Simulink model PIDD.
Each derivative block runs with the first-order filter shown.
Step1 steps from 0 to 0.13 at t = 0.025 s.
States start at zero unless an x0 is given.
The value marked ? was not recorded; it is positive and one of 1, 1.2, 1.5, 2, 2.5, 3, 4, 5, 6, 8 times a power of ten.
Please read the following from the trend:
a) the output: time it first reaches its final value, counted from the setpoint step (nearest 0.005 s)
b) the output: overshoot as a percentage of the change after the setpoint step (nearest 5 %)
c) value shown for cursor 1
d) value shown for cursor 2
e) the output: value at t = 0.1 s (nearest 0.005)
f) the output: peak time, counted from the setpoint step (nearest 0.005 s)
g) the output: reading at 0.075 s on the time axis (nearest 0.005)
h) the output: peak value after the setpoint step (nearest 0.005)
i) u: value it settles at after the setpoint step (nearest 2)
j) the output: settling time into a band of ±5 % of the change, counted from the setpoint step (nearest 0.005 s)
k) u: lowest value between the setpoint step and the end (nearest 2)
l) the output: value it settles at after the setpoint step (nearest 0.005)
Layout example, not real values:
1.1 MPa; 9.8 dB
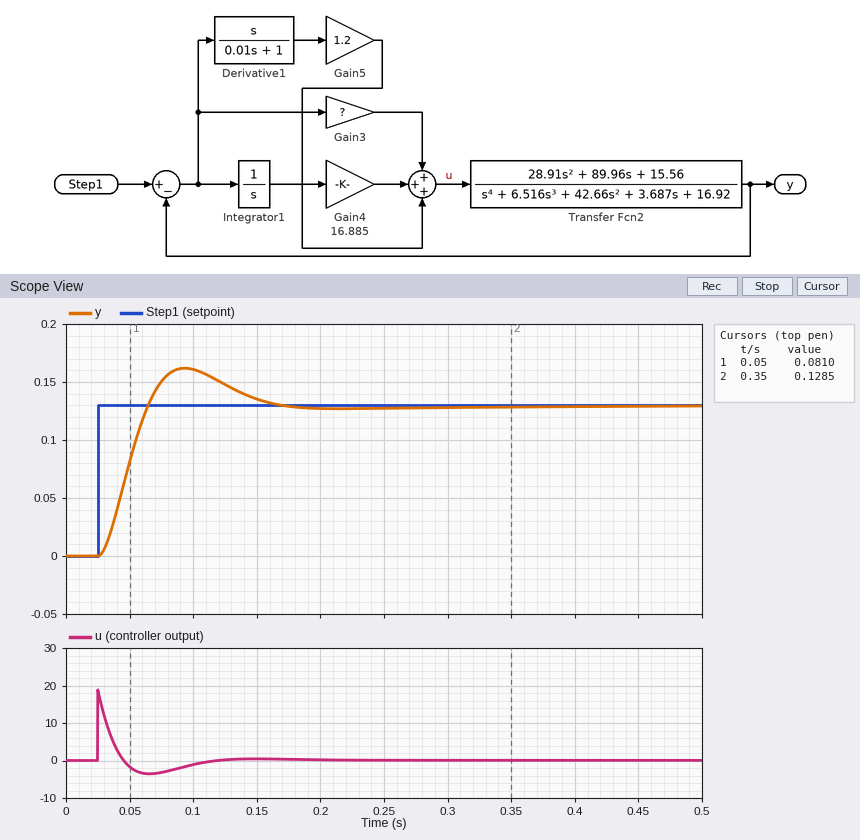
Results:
0.040 s; 25 %; 0.0810; 0.1285; 0.160; 0.070 s; 0.150; 0.160; 0; 0.125 s; -4; 0.130
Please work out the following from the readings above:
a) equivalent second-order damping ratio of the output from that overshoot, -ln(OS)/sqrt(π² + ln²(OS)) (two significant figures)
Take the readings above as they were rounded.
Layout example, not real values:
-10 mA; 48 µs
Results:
0.40
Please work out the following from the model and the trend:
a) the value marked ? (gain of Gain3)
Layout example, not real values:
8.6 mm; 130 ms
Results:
25
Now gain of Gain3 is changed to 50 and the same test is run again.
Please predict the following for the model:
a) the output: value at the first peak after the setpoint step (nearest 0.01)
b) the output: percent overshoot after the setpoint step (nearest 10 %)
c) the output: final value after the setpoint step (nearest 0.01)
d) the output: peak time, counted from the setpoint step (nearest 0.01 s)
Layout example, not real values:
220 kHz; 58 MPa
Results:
0.18; 40 %; 0.13; 0.06 s
